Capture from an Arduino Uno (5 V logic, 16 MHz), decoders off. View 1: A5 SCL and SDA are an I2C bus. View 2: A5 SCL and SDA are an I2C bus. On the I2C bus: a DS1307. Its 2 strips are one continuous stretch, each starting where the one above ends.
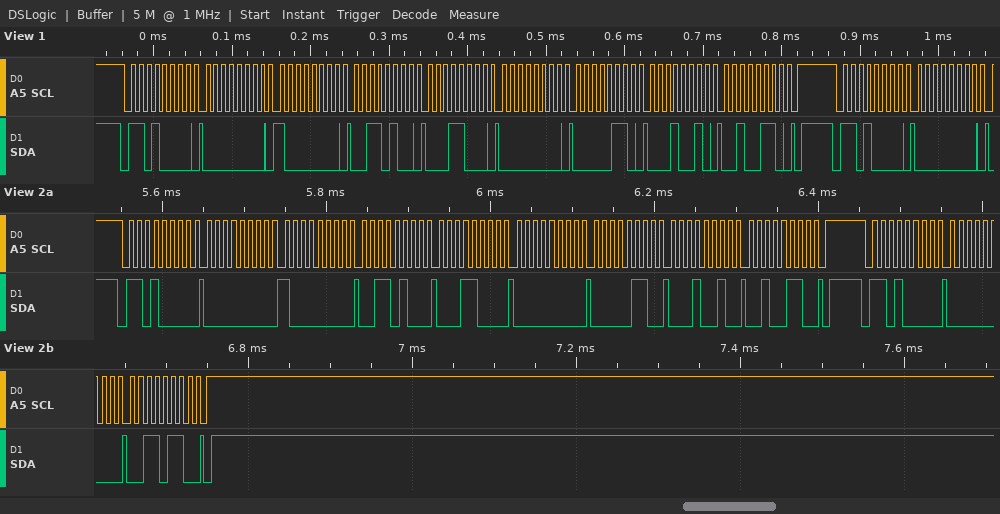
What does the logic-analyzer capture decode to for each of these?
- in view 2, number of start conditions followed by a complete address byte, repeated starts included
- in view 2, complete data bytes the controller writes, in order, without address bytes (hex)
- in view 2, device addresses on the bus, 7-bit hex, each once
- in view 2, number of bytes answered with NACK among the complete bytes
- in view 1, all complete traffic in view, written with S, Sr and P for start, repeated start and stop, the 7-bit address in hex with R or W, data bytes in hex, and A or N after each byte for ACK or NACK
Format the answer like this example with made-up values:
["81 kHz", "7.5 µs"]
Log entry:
["2", "00 80 34 18 00 06 12 26 00 36", "0x68", "0", "S 68W A 00 A 80 A 34 A 18 A 00 A 06 A 12 A 26 A P S 68W A 00 A"]
